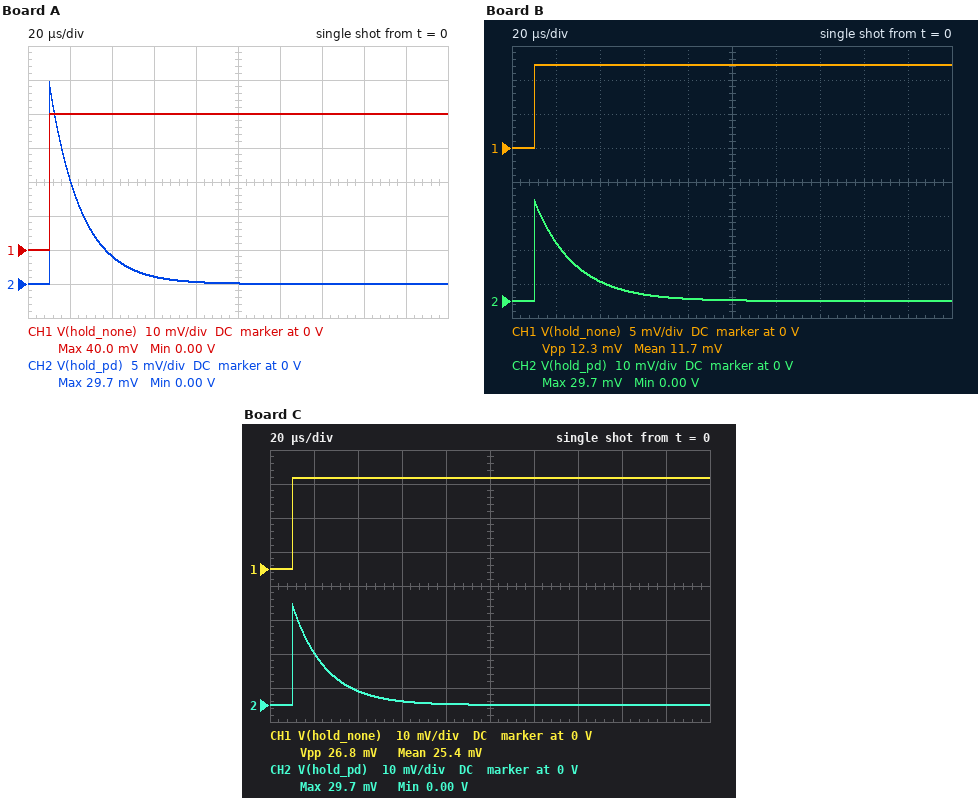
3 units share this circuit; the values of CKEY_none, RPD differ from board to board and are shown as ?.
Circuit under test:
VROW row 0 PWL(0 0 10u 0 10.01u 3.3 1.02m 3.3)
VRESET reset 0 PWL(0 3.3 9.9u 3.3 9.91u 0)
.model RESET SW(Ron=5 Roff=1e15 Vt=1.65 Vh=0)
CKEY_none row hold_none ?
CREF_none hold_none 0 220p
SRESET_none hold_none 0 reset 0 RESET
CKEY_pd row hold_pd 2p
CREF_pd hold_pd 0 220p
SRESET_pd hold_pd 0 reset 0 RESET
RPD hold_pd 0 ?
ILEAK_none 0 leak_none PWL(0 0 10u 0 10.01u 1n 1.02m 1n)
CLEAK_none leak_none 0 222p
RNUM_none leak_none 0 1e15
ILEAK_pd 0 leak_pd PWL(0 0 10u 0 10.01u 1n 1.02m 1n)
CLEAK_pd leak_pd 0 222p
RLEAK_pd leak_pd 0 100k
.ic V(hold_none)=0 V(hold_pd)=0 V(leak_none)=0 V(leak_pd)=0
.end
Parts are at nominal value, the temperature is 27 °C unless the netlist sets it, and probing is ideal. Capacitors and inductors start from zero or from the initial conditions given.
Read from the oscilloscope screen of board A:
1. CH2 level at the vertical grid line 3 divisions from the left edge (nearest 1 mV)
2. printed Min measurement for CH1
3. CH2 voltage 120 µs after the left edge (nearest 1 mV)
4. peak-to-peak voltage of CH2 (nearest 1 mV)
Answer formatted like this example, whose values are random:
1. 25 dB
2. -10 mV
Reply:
1. 1 mV
2. 0.00 V
3. 0 V
4. 30 mV
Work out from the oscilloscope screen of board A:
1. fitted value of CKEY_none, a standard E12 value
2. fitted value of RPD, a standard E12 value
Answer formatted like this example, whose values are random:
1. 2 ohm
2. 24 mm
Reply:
1. 2.7 pF
2. 68 kΩ
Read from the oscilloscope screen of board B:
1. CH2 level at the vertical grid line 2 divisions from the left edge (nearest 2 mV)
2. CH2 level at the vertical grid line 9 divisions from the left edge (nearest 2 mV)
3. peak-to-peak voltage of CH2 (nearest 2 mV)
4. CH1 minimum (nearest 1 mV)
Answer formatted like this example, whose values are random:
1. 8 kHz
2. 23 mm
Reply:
1. 6 mV
2. 0 V
3. 30 mV
4. 0 V
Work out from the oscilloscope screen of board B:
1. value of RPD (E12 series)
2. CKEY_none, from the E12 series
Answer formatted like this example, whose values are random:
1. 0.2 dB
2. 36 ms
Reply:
1. 82 kΩ
2. 820 fF
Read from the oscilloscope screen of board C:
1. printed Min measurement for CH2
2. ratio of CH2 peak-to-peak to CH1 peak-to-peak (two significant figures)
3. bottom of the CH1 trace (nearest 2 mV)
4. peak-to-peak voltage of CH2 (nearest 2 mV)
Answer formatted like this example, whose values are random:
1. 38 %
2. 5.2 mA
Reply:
1. 0.00 V
2. 1.1
3. 0 V
4. 30 mV
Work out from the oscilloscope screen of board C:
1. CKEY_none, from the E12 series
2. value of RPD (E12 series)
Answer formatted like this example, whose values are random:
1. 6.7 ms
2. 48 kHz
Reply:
1. 1.8 pF
2. 68 kΩ
